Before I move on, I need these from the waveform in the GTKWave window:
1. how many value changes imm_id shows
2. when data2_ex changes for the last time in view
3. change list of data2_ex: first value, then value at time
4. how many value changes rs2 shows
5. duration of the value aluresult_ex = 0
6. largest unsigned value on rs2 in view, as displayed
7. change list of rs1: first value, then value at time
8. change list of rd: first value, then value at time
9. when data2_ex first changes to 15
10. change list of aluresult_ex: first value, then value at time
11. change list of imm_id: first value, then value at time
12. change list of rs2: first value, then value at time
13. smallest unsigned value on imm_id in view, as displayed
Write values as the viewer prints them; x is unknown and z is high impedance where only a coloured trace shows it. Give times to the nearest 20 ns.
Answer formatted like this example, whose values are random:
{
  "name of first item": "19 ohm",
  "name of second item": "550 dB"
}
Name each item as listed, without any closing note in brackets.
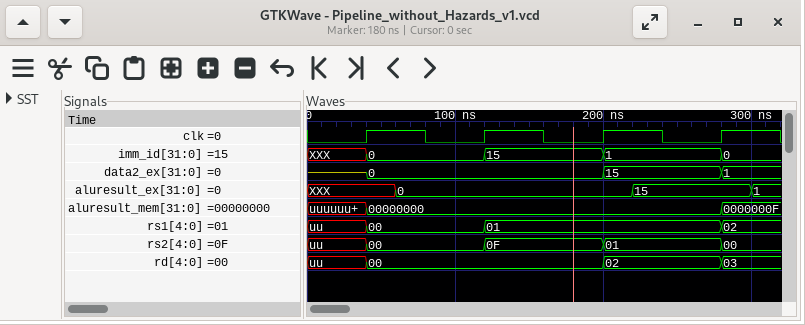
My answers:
{
  "how many value changes imm_id shows": "4",
  "when data2_ex changes for the last time in view": "280 ns",
  "change list of data2_ex: first value, then value at time": "z, 0 at 40 ns, 15 at 200 ns, 1 at 280 ns",
  "how many value changes rs2 shows": "4",
  "duration of the value aluresult_ex = 0": "160 ns",
  "largest unsigned value on rs2 in view, as displayed": "0F",
  "change list of rs1: first value, then value at time": "uu, 00 at 40 ns, 01 at 120 ns, 02 at 280 ns",
  "change list of rd: first value, then value at time": "uu, 00 at 40 ns, 02 at 200 ns, 03 at 280 ns",
  "when data2_ex first changes to 15": "200 ns",
  "change list of aluresult_ex: first value, then value at time": "XXX, 0 at 60 ns, 15 at 220 ns, 1 at 300 ns",
  "change list of imm_id: first value, then value at time": "XXX, 0 at 40 ns, 15 at 120 ns, 1 at 200 ns, 0 at 280 ns",
  "change list of rs2: first value, then value at time": "uu, 00 at 40 ns, 0F at 120 ns, 01 at 200 ns, 00 at 280 ns",
  "smallest unsigned value on imm_id in view, as displayed": "0"
}
